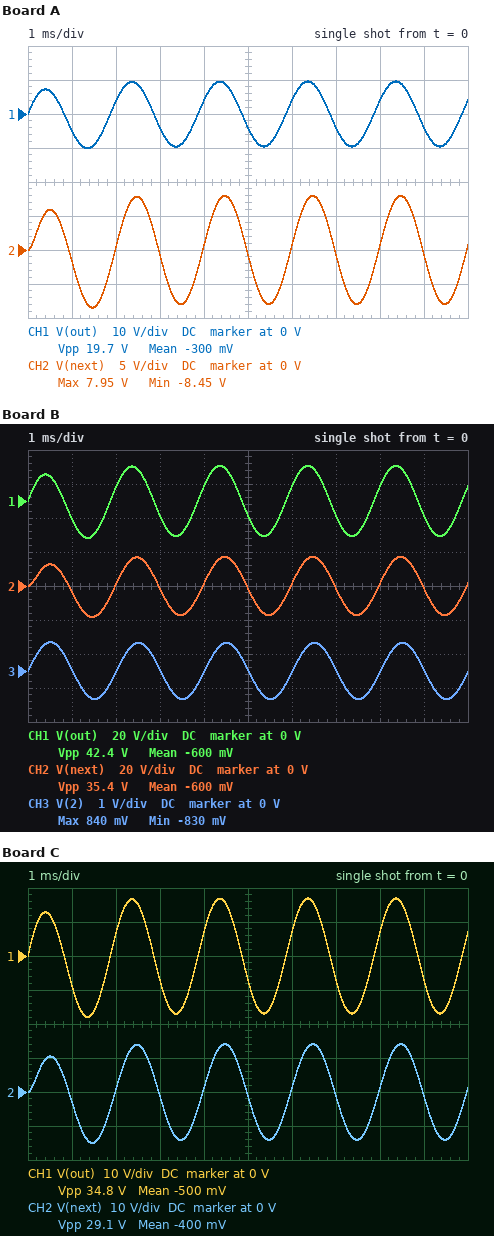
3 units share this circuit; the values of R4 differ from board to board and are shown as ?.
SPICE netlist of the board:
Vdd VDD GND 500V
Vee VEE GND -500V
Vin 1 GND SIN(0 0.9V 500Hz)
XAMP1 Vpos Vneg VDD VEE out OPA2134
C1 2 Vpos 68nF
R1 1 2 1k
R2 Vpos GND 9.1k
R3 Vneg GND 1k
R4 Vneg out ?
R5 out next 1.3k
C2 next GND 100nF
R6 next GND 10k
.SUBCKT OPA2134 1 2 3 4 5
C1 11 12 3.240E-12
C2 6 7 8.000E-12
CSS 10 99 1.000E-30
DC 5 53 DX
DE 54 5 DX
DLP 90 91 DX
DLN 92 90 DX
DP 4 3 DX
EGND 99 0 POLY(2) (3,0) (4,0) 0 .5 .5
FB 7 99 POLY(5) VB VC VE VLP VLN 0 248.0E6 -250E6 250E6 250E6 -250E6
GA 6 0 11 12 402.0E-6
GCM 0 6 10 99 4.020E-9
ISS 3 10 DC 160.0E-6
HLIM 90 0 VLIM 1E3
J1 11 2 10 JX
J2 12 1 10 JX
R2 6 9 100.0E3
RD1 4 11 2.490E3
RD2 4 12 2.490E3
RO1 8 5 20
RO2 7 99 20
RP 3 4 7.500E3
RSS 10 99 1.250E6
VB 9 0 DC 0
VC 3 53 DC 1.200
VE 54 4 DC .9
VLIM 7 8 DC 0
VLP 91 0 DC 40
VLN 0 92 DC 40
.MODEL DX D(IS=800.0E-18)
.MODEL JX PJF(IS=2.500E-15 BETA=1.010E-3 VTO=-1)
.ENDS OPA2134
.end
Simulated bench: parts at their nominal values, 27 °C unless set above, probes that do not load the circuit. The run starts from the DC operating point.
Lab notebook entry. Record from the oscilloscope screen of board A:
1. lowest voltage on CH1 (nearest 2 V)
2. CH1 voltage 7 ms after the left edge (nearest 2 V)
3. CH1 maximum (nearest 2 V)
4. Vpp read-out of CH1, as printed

-10 V
-4 V
10 V
19.7 V
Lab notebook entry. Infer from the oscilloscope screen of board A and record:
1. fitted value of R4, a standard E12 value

12 kΩ
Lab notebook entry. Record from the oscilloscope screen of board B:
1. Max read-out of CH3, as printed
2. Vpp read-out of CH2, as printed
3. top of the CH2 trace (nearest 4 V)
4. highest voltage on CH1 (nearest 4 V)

840 mV
35.4 V
16 V
20 V
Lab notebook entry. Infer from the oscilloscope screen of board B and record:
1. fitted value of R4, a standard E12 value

27 kΩ
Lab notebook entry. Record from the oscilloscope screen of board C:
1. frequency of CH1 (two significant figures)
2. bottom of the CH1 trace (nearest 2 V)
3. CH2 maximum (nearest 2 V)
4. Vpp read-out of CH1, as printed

500 Hz
-18 V
14 V
34.8 V
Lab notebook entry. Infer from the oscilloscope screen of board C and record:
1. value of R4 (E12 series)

22 kΩ
